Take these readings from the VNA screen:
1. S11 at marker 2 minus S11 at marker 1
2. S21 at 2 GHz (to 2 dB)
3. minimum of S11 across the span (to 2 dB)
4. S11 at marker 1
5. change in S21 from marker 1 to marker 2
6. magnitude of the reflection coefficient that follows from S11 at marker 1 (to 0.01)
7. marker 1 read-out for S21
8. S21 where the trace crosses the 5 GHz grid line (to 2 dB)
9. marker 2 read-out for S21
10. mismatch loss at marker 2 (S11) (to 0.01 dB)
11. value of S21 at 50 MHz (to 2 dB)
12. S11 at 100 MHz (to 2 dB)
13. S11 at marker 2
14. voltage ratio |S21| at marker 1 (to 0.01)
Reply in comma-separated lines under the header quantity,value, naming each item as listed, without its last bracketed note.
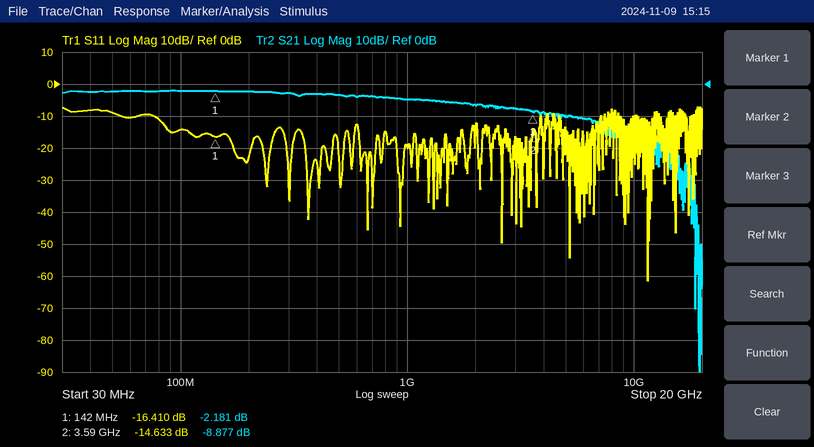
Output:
quantity,value
S11 at marker 2 minus S11 at marker 1,1.777 dB
S21 at 2 GHz,-6 dB
minimum of S11 across the span,-62 dB
S11 at marker 1,-16.410 dB
change in S21 from marker 1 to marker 2,-6.696 dB
magnitude of the reflection coefficient that follows from S11 at marker 1,0.15
marker 1 read-out for S21,-2.181 dB
S21 where the trace crosses the 5 GHz grid line,-10 dB
marker 2 read-out for S21,-8.877 dB
mismatch loss at marker 2 (S11),0.15 dB
value of S21 at 50 MHz,-2 dB
S11 at 100 MHz,-14 dB
S11 at marker 2,-14.633 dB
voltage ratio |S21| at marker 1,0.78
